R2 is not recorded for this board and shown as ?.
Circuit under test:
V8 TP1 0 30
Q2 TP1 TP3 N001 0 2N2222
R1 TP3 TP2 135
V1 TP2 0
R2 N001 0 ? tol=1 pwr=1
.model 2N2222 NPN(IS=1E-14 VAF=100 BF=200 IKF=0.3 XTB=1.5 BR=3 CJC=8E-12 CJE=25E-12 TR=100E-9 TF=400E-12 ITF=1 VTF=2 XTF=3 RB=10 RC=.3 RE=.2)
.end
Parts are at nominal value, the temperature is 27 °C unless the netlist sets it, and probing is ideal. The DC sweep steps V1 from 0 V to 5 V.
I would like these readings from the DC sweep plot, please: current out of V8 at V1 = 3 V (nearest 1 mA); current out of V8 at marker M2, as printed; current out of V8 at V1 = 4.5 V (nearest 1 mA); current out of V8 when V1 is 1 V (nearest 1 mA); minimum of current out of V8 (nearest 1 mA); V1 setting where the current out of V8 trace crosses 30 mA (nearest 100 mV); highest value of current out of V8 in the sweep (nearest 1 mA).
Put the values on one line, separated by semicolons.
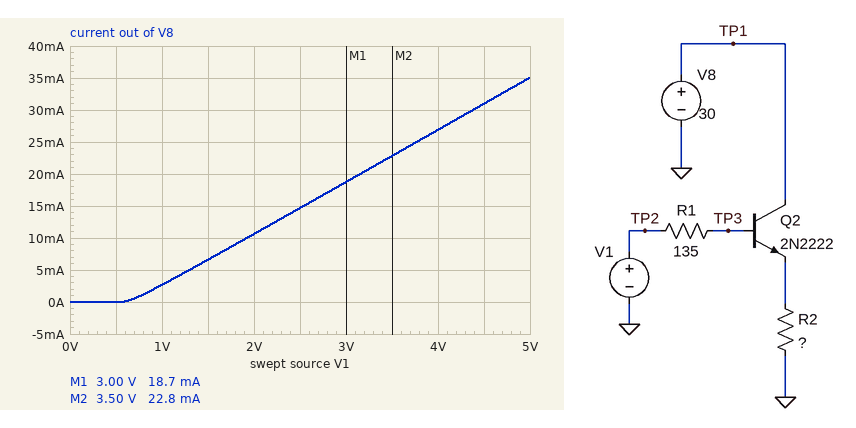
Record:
19 mA; 22.8 mA; 31 mA; 3 mA; 0 A; 4.4 V; 35 mA
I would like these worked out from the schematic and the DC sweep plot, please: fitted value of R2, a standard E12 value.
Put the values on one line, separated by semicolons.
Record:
120 Ω
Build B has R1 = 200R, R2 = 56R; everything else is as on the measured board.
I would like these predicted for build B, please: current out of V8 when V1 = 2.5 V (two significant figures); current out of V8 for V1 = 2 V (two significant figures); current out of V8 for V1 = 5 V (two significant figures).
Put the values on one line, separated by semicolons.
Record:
31 mA; 22 mA; 74 mA
